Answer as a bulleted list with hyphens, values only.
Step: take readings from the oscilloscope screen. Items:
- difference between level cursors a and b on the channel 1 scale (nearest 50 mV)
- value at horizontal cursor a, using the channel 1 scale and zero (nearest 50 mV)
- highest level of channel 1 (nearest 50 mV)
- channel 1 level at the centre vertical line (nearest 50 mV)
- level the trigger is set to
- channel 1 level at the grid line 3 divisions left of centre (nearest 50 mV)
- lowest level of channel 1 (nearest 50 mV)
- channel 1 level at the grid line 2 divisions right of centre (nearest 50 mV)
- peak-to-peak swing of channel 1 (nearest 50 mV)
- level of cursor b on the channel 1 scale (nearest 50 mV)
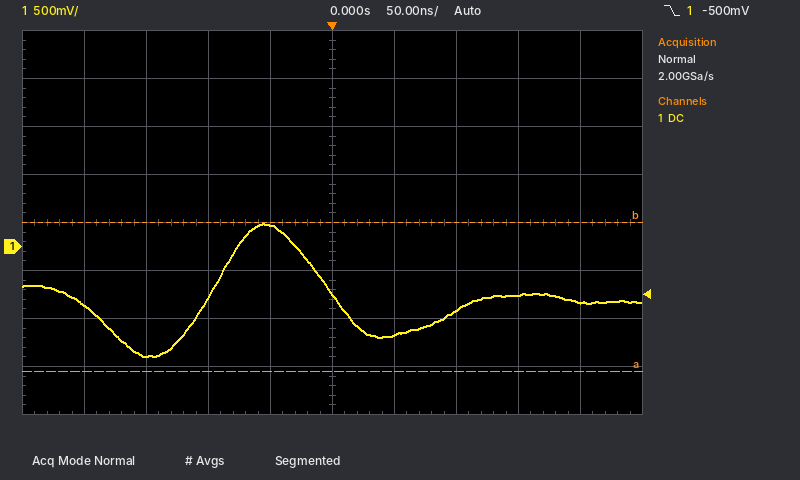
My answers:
- 1.55 V
- -1.30 V
- 250 mV
- -500 mV
- -500 mV
- -1.15 V
- -1.15 V
- -650 mV
- 1.40 V
- 250 mV
